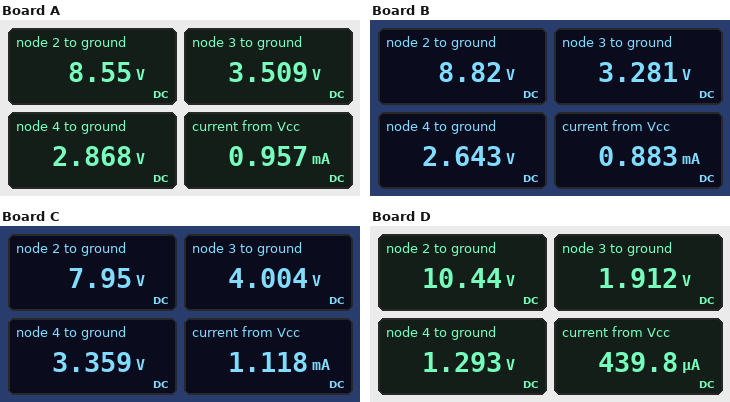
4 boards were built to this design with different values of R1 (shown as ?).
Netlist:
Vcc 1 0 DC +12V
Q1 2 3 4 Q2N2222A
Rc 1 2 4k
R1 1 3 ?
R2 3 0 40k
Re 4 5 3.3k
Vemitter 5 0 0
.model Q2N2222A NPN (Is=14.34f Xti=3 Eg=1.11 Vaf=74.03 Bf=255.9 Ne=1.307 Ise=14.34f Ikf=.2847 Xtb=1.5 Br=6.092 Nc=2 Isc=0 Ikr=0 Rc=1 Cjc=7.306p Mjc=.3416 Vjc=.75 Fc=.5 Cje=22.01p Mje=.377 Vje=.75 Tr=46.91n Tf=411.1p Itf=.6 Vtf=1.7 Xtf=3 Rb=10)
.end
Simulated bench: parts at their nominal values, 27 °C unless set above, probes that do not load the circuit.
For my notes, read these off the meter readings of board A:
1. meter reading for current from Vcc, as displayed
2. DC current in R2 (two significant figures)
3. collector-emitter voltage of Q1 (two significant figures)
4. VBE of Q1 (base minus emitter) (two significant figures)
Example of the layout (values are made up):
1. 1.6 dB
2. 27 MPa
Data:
1. 0.957 mA
2. 88 µA
3. 5.7 V
4. 640 mV
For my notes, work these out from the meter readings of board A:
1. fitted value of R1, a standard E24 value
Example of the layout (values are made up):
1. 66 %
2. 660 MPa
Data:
1. 91 kΩ
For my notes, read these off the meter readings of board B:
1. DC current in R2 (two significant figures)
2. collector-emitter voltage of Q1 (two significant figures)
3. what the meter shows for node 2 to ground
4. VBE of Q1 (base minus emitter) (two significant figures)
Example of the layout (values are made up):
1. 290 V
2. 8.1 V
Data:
1. 82 µA
2. 6.2 V
3. 8.82 V
4. 640 mV
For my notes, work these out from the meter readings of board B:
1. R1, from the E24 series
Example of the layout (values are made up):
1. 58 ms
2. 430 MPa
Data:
1. 100 kΩ
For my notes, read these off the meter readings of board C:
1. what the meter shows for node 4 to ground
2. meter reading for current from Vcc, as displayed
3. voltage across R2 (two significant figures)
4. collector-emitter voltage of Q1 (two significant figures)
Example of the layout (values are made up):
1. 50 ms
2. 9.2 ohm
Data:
1. 3.359 V
2. 1.118 mA
3. 4.0 V
4. 4.6 V
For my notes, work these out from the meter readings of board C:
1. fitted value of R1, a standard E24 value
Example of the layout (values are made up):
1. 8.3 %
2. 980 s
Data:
1. 75 kΩ
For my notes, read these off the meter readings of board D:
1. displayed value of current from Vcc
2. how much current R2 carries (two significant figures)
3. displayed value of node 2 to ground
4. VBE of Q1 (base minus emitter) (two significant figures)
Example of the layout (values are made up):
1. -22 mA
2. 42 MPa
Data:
1. 439.8 µA
2. 48 µA
3. 10.44 V
4. 620 mV
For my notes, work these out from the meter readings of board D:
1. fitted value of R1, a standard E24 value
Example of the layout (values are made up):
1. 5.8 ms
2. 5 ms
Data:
1. 200 kΩ
